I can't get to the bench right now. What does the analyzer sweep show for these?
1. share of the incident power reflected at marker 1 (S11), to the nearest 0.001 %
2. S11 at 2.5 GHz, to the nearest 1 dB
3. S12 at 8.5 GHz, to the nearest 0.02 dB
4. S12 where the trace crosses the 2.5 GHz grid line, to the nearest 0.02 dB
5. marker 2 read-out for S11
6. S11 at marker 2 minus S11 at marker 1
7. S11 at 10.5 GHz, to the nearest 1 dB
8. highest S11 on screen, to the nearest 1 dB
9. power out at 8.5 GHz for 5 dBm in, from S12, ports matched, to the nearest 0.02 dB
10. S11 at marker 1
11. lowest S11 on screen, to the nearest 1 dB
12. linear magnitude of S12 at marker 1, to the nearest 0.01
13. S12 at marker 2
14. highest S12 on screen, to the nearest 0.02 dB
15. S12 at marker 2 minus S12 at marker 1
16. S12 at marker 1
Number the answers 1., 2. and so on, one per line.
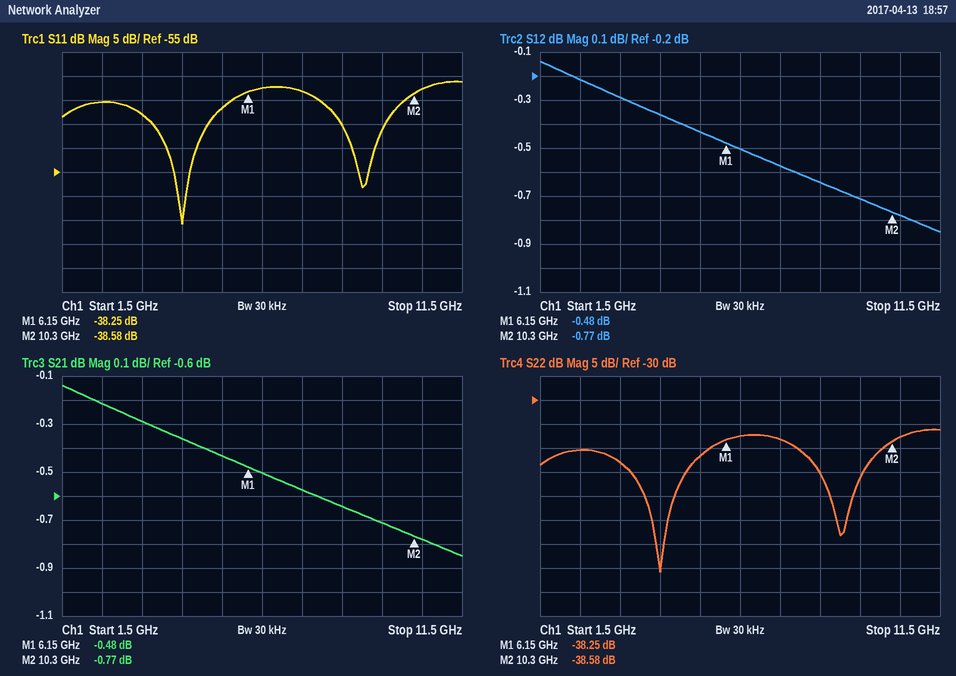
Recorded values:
1. 0.015 %
2. -40 dB
3. -0.64 dB
4. -0.22 dB
5. -38.58 dB
6. -0.33 dB
7. -38 dB
8. -36 dB
9. 4.36 dBm
10. -38.25 dB
11. -66 dB
12. 0.95
13. -0.77 dB
14. -0.14 dB
15. -0.29 dB
16. -0.48 dB
